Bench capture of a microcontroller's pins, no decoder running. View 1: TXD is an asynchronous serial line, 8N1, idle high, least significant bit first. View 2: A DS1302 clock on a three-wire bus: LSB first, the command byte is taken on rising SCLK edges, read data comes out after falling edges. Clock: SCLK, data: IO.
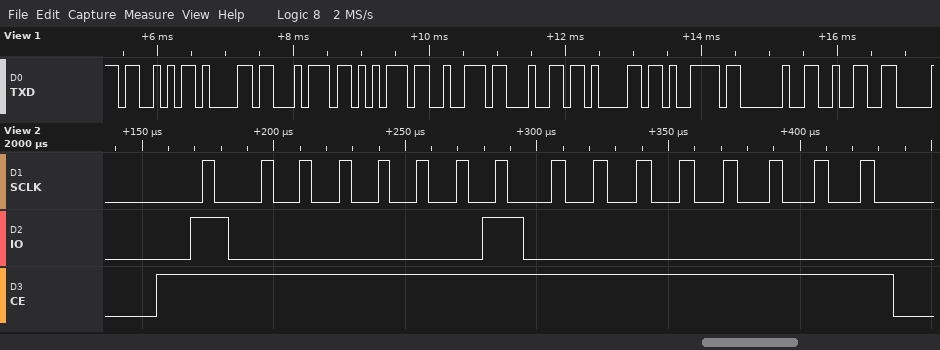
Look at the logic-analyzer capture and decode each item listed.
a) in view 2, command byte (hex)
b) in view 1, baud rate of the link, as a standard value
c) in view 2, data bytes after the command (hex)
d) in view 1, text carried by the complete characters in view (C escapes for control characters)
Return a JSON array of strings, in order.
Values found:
["0x81", "9600 baud", "00", "\"Saturday 2\""]
